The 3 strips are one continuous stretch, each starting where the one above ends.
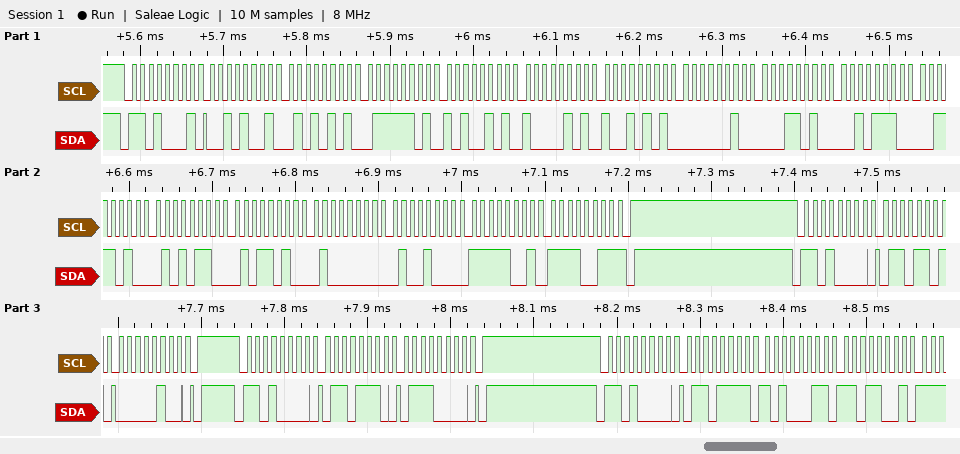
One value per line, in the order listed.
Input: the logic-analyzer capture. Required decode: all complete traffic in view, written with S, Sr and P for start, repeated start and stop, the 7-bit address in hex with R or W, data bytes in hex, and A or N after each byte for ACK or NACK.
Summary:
S 68R A 29 A 55 A 7D A A5 A 85 A 95 A 02 A 1A A 2E A 3A A 56 A 5A A 40 A 48 A F9 A F3 N P S 68W A 6D A 04 A P S 68W A 6E A 70 A P S 68W A 6F A A3 A D9 A
